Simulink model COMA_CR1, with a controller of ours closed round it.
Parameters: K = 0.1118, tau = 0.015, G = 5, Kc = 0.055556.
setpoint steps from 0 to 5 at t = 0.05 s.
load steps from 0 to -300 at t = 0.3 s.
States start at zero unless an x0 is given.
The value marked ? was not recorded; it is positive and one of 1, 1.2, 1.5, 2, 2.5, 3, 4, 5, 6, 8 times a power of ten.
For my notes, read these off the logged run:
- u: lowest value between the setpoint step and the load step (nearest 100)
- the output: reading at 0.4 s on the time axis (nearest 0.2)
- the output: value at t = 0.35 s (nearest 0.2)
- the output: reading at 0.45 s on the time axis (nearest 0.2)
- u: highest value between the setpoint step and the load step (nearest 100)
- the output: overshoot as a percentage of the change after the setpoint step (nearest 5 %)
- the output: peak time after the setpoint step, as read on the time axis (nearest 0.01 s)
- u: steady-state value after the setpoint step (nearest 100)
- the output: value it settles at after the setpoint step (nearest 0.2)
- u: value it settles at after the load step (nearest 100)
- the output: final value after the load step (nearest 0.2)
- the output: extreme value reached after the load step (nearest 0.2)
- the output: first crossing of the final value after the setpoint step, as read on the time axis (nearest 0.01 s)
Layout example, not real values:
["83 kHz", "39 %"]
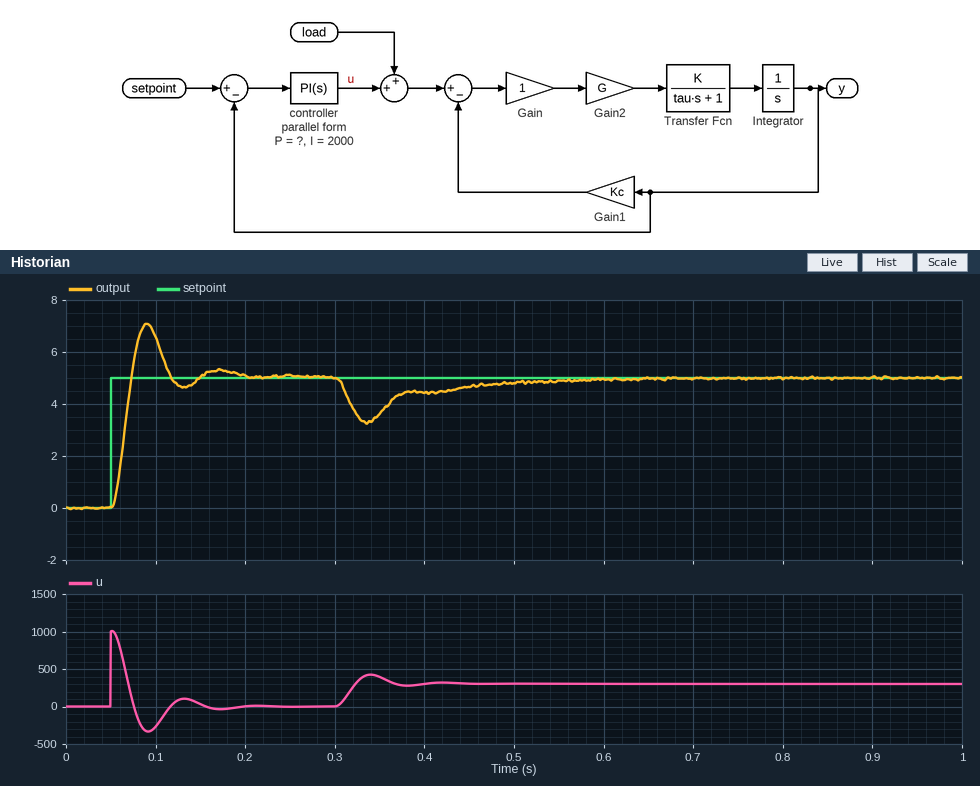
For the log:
["-300", "4.4", "3.6", "4.6", "1000", "40 %", "0.09 s", "0", "5.0", "300", "5.0", "3.2", "0.07 s"]
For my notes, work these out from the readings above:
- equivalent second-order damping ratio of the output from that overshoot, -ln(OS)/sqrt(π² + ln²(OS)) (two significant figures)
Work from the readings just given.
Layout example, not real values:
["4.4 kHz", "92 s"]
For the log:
["0.28"]
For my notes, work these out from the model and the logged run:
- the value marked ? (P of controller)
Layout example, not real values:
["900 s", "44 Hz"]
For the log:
["200"]
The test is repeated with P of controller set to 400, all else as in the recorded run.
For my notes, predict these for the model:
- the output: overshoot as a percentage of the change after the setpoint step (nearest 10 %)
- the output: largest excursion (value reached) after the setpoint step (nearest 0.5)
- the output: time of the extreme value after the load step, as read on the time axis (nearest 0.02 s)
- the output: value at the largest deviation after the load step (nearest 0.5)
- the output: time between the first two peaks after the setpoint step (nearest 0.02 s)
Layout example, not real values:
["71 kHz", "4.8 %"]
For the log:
["50 %", "7.5", "0.32 s", "4.0", "0.06 s"]
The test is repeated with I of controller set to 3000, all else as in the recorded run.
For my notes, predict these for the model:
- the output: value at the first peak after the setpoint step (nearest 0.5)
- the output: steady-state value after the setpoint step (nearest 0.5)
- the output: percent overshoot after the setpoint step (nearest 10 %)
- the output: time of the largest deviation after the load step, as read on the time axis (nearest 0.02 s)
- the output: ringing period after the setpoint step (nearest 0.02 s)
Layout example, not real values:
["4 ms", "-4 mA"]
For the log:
["7.5", "5.0", "50 %", "0.34 s", "0.08 s"]
